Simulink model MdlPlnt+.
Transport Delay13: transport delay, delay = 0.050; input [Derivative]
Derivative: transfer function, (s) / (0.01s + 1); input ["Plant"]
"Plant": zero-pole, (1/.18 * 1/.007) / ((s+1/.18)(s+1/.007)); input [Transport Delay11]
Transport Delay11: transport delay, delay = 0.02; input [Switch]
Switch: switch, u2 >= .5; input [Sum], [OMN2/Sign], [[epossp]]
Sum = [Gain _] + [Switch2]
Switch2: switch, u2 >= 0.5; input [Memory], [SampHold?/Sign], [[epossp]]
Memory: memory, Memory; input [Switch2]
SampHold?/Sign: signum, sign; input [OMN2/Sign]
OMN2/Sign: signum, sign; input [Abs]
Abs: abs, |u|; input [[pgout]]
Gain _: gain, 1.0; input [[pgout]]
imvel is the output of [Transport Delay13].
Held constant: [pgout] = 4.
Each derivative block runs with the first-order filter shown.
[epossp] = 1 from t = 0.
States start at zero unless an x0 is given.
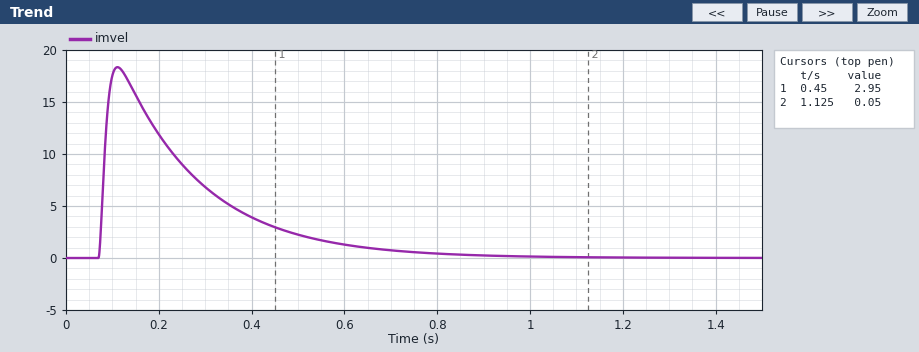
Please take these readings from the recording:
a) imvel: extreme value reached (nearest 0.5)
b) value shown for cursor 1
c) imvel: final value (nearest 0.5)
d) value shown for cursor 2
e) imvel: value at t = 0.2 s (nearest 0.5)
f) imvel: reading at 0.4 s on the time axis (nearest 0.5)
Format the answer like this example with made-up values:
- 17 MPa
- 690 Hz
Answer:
- 18.5
- 2.95
- 0.0
- 0.05
- 12.0
- 4.0
